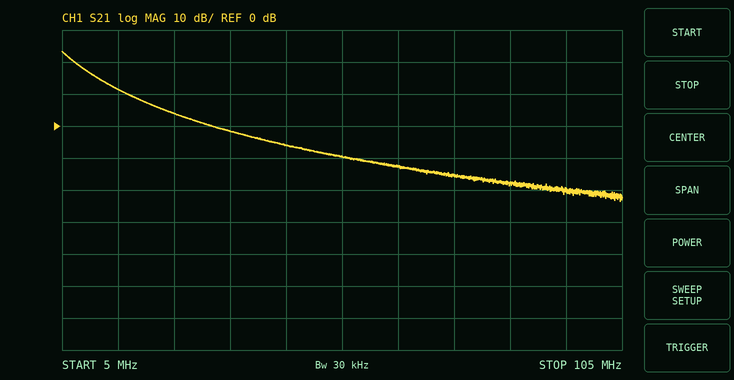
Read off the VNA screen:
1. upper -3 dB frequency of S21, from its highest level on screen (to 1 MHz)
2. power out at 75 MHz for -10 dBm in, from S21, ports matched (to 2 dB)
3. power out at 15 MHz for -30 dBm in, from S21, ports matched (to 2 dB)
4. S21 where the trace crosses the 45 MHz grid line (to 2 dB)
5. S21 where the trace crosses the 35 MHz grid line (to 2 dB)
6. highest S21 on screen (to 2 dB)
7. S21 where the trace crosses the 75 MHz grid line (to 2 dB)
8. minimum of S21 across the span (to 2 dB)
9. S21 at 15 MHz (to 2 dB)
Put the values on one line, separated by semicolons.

7 MHz; -26 dBm; -18 dBm; -6 dB; -2 dB; 24 dB; -16 dB; -24 dB; 12 dB
